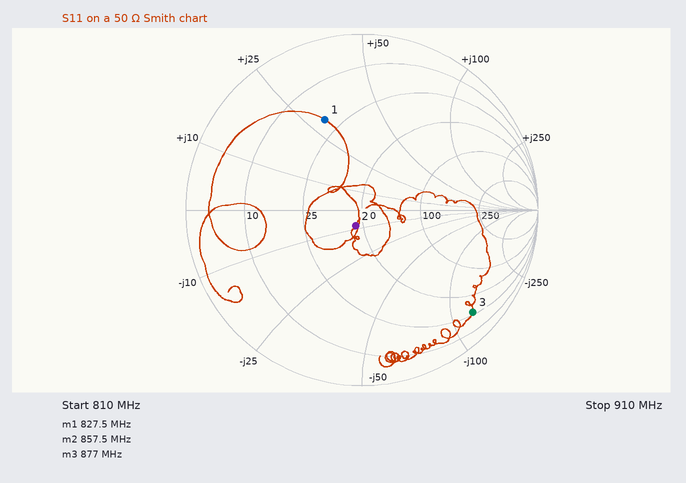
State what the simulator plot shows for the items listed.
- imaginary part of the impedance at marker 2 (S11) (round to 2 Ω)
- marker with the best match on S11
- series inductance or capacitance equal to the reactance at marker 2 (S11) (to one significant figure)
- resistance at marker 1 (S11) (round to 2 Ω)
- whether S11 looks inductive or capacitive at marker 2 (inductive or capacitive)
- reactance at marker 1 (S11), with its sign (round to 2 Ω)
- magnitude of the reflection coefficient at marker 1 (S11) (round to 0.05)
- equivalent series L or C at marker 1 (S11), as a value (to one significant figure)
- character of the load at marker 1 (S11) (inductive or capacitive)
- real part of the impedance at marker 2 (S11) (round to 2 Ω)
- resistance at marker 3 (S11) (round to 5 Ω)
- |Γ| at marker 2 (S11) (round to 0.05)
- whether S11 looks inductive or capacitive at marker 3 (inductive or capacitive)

-8 Ω
marker 2
20 pF
20 Ω
capacitive
+30 Ω
0.55
6 nH
inductive
46 Ω
30 Ω
0.10
capacitive
